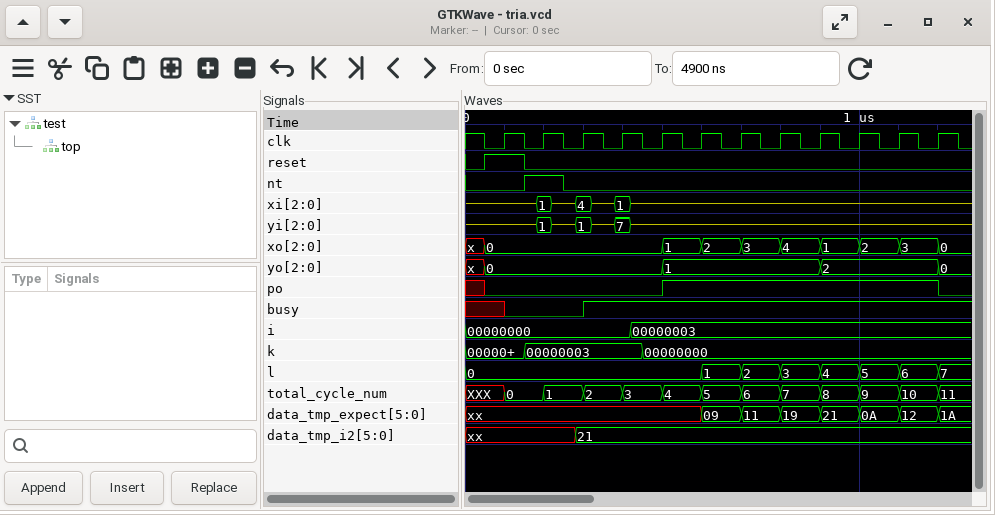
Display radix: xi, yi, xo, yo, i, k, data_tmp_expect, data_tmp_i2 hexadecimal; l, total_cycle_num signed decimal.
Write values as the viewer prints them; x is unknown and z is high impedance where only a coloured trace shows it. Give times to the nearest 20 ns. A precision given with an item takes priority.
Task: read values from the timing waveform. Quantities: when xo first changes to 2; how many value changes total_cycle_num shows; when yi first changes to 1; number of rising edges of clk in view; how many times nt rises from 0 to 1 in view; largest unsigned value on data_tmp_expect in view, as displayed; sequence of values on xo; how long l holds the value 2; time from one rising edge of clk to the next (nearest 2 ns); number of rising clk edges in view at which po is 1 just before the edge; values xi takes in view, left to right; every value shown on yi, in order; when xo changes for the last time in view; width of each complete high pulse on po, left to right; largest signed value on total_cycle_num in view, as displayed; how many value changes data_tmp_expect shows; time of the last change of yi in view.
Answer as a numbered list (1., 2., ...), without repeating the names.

1. 600 ns
2. 12
3. 180 ns
4. 12
5. 1
6. 21
7. x, 0, 1, 2, 3, 4, 1, 2, 3, 0
8. 100 ns
9. 100 ns
10. 7
11. z, 1, z, 4, z, 1, z
12. z, 1, z, 1, z, 7, z
13. 1200 ns
14. 700 ns
15. 11
16. 7
17. 420 ns
